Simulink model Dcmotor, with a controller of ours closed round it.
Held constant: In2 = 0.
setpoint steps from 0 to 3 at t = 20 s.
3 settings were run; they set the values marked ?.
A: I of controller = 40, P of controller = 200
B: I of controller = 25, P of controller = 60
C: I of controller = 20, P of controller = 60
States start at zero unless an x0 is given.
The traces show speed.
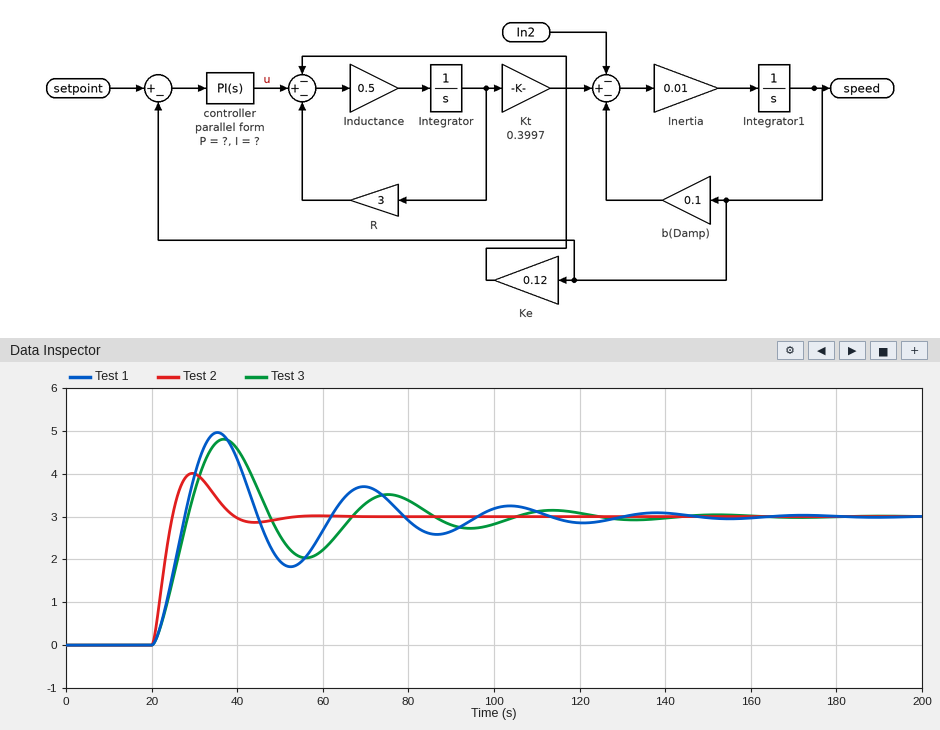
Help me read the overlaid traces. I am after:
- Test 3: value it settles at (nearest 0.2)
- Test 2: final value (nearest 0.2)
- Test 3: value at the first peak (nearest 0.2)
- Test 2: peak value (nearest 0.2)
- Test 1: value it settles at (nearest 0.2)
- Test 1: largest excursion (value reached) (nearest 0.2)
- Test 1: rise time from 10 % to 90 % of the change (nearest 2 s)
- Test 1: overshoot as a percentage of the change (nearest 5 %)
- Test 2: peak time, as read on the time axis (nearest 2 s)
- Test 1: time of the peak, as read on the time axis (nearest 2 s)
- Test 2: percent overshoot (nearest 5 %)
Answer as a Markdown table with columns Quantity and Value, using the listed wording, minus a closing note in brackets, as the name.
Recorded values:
| Quantity | Value |
|---|---|
| Test 3: value it settles at | 3.0 |
| Test 2: final value | 3.0 |
| Test 3: value at the first peak | 4.8 |
| Test 2: peak value | 4.0 |
| Test 1: value it settles at | 3.0 |
| Test 1: largest excursion (value reached) | 5.0 |
| Test 1: rise time from 10 % to 90 % of the change | 6 s |
| Test 1: overshoot as a percentage of the change | 65 % |
| Test 2: peak time, as read on the time axis | 30 s |
| Test 1: time of the peak, as read on the time axis | 36 s |
| Test 2: percent overshoot | 35 % |
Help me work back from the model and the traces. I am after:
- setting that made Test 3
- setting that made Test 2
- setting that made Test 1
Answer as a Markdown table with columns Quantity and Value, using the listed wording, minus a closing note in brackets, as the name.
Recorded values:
| Quantity | Value |
|---|---|
| setting that made Test 3 | C |
| setting that made Test 2 | A |
| setting that made Test 1 | B |
